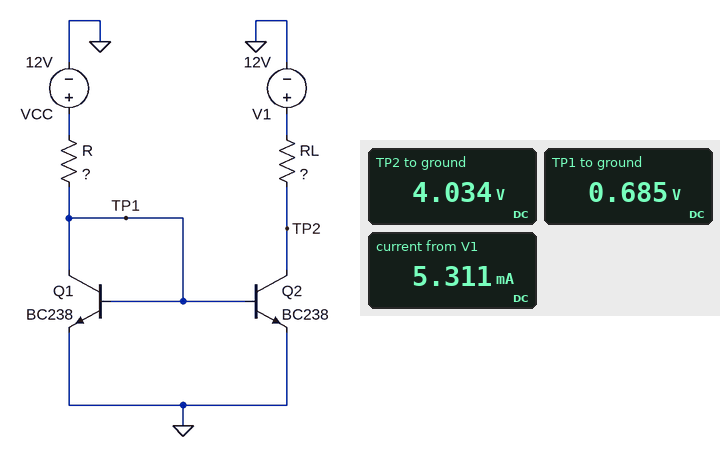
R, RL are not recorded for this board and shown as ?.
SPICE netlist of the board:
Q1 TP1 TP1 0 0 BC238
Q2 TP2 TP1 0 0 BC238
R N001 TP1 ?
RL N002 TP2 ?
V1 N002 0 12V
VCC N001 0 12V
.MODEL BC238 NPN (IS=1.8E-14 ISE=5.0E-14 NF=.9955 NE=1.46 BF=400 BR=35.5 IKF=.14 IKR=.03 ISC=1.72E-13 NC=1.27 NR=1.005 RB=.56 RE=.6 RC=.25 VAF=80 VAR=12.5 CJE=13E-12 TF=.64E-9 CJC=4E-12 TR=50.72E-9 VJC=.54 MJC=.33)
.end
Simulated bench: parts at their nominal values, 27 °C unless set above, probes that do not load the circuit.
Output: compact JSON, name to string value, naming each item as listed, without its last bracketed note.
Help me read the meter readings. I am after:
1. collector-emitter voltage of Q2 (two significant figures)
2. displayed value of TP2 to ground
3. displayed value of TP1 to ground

{"collector-emitter voltage of Q2": "4.0 V", "displayed value of TP2 to ground": "4.034 V", "displayed value of TP1 to ground": "0.685 V"}
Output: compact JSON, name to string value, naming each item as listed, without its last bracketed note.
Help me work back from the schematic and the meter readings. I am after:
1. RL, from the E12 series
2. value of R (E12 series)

{"RL, from the E12 series": "1.5 kΩ", "value of R": "2.2 kΩ"}
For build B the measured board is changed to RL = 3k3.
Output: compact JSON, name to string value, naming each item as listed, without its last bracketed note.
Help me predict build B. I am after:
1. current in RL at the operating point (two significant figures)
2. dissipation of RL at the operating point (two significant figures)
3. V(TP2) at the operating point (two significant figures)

{"current in RL at the operating point": "3.6 mA", "dissipation of RL at the operating point": "43 mW", "V(TP2) at the operating point": "34 mV"}
